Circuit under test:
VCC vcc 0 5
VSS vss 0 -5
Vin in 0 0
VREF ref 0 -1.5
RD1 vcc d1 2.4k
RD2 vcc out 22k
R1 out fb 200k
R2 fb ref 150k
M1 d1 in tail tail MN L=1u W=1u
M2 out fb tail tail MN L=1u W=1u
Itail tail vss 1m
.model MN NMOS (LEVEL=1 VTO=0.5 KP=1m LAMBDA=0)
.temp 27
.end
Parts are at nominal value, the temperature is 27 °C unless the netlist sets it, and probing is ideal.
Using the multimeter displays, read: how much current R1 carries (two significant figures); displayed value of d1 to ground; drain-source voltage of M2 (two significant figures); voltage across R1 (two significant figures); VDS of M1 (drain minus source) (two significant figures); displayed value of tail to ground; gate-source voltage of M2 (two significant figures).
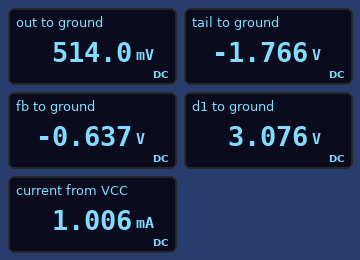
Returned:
5.8 µA
3.076 V
2.3 V
1.2 V
4.8 V
-1.766 V
1.1 V
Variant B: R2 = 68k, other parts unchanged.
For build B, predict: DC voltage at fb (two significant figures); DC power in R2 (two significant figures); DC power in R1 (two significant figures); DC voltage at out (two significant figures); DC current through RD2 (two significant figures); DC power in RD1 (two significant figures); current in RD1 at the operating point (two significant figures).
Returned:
-750 mV
8.2 µW
24 µW
1.4 V
160 µA
1.7 mW
850 µA
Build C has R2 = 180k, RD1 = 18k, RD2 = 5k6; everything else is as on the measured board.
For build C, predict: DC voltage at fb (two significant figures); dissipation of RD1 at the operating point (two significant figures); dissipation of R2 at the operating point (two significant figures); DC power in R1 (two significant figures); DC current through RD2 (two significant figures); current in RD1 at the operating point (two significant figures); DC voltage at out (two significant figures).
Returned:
-140 mV
2.3 mW
10 µW
11 µW
650 µA
360 µA
1.4 V
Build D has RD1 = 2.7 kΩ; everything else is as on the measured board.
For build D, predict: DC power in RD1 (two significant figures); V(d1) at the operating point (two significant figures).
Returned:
1.7 mW
2.8 V
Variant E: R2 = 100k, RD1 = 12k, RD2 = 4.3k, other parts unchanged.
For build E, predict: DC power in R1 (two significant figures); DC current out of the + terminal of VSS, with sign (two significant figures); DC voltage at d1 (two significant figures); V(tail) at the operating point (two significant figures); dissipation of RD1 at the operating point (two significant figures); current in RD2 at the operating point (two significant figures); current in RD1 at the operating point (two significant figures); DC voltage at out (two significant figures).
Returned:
40 µW
-1.0 mA
-930 mV
-1.6 V
2.9 mW
520 µA
490 µA
2.8 V
